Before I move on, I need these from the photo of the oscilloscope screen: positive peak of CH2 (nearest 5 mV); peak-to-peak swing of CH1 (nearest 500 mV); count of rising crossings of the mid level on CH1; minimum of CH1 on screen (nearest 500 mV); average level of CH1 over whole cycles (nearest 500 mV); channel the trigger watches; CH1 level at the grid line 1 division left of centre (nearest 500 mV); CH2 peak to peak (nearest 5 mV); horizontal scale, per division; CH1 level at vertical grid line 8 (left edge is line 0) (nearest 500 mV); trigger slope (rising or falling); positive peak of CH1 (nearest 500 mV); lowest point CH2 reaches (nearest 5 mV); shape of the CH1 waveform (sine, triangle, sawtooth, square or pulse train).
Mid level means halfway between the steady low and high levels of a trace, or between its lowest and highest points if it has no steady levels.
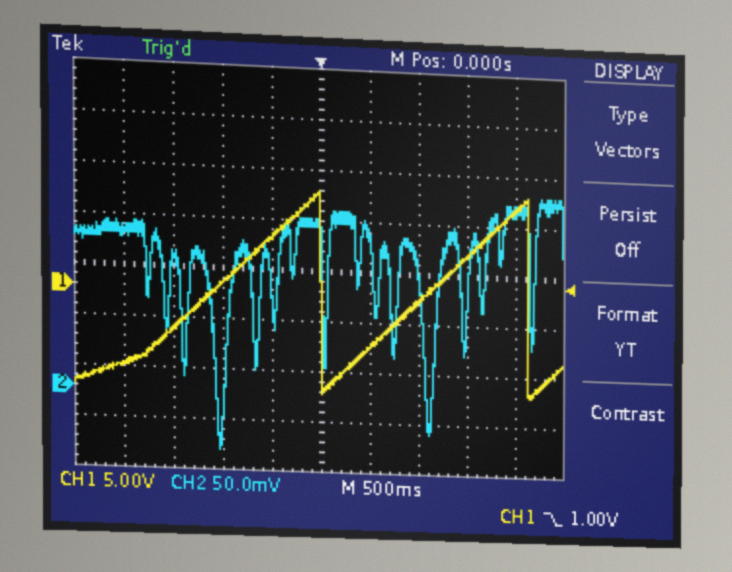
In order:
200 mV
20.0 V
2
-10.0 V
0.0 V
CH1
5.5 V
260 mV
500 ms
4.0 V
falling
10.0 V
-60 mV
sawtooth
